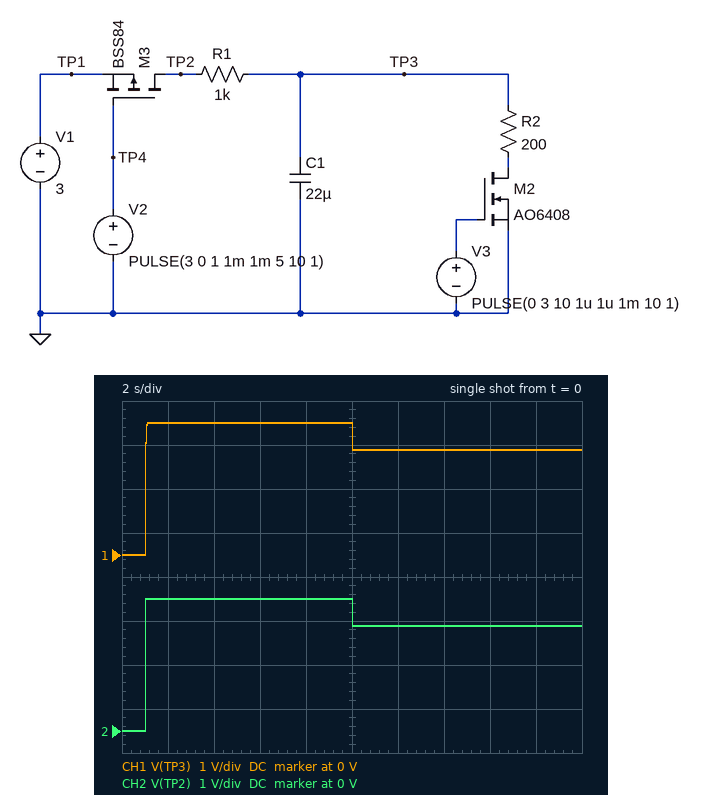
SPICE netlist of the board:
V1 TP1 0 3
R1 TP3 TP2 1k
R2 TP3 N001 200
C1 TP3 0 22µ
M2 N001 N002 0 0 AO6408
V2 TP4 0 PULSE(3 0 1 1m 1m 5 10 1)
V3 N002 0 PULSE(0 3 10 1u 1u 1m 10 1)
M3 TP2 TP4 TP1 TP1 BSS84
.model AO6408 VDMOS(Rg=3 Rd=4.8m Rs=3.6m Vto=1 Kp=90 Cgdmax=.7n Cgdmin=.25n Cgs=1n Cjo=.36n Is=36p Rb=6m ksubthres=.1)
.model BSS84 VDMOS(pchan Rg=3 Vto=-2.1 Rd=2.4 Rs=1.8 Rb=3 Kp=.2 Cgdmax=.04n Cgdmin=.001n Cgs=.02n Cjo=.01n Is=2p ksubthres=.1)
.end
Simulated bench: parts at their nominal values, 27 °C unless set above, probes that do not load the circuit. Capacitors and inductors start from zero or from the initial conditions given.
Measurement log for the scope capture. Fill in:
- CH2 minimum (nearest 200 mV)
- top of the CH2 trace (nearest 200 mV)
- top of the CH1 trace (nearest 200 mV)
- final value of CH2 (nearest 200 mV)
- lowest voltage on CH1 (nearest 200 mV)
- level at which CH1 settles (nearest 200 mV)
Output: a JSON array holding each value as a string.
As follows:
["0 V", "3.0 V", "3.0 V", "2.4 V", "0 V", "2.4 V"]
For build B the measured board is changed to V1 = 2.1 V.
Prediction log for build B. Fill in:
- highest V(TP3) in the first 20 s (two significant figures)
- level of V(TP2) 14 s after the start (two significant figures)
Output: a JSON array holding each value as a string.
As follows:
["2.1 V", "1.7 V"]
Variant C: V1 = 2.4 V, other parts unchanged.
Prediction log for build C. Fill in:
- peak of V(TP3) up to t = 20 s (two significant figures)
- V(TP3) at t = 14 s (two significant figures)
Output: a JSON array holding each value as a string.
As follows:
["2.4 V", "1.9 V"]
